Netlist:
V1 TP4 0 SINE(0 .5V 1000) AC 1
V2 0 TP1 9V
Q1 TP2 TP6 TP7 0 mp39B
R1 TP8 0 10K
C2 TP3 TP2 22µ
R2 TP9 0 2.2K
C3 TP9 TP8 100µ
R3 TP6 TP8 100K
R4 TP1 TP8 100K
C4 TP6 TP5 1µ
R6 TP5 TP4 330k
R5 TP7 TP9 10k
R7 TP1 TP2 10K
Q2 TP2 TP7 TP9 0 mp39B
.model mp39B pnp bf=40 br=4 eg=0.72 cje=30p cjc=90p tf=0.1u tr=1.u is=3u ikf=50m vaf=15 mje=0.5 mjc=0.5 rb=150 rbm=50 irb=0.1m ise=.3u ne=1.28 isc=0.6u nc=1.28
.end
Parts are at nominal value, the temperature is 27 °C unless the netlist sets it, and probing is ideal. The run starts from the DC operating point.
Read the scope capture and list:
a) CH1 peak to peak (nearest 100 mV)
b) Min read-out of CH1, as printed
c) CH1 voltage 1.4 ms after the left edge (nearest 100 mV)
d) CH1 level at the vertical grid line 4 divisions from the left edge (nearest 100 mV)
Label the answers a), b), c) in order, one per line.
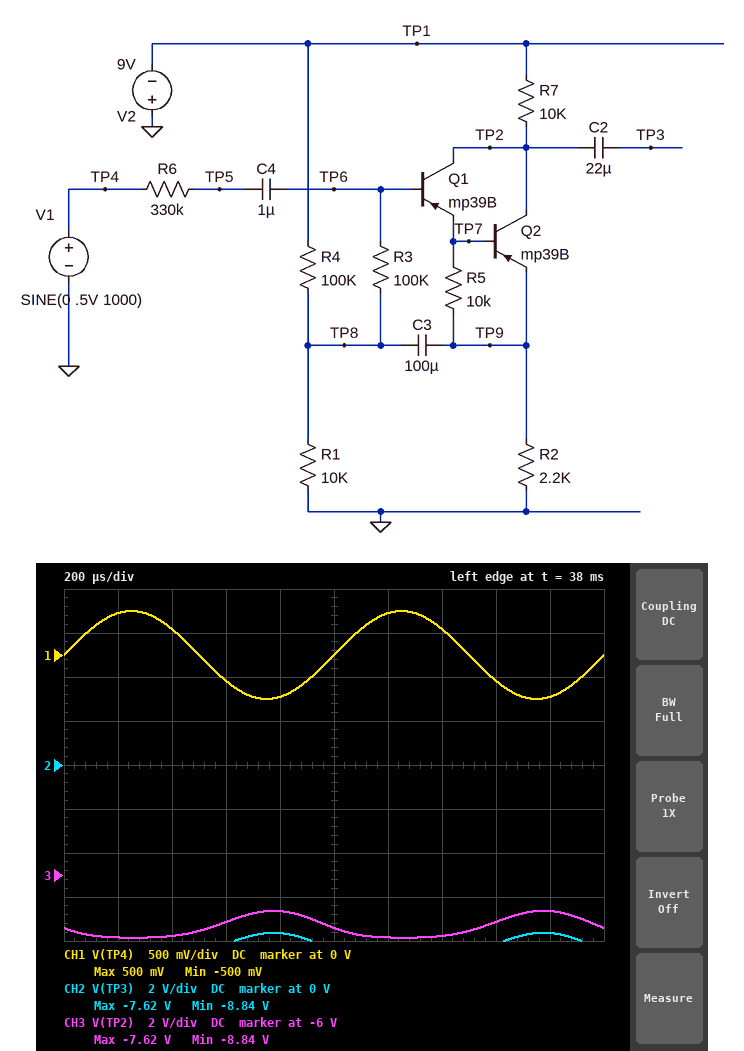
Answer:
a) 1.0 V
b) -500 mV
c) 300 mV
d) -500 mV
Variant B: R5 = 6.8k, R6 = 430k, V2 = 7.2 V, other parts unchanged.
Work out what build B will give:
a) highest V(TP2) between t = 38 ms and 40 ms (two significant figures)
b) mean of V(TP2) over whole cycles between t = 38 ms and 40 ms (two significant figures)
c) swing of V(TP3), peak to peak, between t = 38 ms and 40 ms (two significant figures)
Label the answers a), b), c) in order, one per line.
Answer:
a) -6.2 V
b) -6.7 V
c) 870 mV
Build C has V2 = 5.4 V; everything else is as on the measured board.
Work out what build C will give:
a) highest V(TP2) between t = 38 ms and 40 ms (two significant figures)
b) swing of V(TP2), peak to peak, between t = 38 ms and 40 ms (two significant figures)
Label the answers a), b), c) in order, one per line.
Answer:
a) -4.2 V
b) 1.0 V
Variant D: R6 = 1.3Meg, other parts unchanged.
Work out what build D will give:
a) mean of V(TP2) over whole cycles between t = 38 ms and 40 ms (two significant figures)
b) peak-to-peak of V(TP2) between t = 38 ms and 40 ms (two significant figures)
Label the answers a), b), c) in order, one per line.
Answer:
a) -8.1 V
b) 650 mV
